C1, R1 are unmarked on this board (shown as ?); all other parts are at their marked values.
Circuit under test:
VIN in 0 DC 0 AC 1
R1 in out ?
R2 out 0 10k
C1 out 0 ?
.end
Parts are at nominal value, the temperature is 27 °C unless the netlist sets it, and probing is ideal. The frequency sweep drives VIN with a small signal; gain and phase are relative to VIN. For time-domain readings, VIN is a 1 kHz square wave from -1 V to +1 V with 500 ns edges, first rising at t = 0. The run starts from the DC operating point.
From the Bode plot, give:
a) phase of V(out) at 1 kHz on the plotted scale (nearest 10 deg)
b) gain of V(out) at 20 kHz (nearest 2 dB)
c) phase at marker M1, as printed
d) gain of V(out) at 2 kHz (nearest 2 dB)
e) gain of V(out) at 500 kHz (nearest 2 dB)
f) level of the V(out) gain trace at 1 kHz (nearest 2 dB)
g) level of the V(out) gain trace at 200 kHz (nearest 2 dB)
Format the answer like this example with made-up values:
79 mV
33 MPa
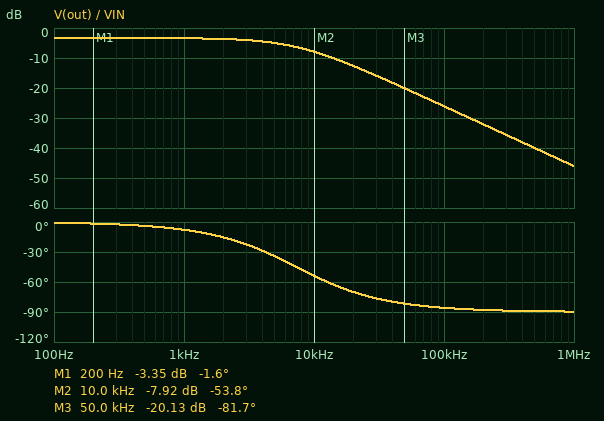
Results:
-10 deg
-12 dB
-1.6 deg
-4 dB
-40 dB
-4 dB
-32 dB
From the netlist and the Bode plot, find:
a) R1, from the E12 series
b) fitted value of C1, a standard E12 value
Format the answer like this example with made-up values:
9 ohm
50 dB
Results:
4.7 kΩ
6.8 nF
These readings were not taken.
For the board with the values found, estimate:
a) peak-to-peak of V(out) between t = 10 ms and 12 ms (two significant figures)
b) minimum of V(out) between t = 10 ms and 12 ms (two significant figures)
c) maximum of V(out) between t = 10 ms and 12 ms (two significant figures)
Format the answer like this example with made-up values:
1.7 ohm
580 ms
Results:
1.4 V
-680 mV
680 mV
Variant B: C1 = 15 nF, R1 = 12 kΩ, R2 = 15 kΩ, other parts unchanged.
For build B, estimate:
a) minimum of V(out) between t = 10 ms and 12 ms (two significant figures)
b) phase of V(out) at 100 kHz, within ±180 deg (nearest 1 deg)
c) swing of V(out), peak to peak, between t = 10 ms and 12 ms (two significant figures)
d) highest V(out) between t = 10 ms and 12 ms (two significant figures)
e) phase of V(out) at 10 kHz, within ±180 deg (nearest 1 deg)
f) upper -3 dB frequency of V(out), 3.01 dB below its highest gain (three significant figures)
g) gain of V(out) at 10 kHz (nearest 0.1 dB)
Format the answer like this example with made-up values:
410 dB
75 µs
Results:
-550 mV
-89 deg
1.1 V
550 mV
-81 deg
1.59 kHz
-21.2 dB
